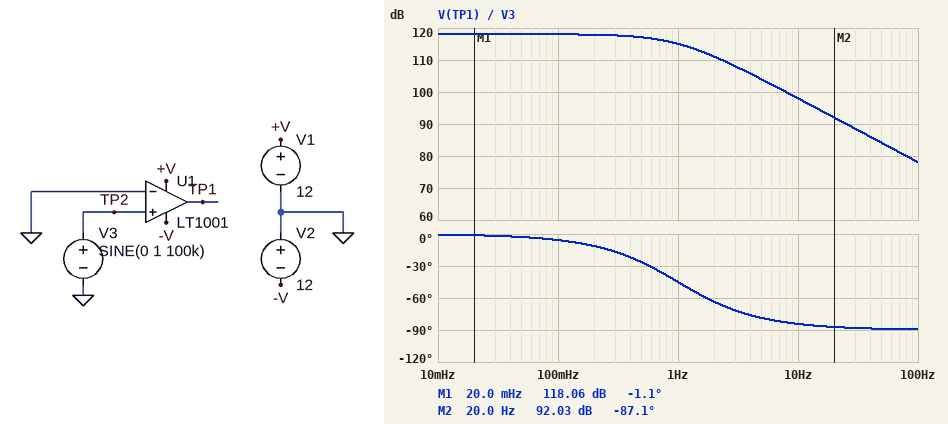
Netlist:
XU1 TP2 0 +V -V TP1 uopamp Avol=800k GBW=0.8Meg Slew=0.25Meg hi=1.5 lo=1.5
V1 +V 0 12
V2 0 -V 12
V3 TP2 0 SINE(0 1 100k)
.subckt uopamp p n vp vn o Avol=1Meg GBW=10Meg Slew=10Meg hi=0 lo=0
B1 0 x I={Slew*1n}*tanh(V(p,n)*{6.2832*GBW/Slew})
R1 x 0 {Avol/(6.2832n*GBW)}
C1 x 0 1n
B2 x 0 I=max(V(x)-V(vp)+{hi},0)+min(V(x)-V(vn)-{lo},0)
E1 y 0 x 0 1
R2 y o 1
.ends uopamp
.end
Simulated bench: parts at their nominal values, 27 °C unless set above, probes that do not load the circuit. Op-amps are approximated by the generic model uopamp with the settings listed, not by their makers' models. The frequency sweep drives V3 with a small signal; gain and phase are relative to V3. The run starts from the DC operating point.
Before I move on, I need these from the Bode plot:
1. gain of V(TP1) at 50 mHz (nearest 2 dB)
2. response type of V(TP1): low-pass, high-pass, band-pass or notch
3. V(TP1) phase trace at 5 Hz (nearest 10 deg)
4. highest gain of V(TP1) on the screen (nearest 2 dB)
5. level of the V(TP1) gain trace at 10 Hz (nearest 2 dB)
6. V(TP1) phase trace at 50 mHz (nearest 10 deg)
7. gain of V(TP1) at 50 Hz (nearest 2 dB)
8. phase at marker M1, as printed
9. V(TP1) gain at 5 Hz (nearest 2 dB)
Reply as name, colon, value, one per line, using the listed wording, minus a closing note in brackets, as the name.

gain of V(TP1) at 50 mHz: 118 dB
response type of V(TP1): low-pass, high-pass, band-pass or notch: low-pass
V(TP1) phase trace at 5 Hz: -80 deg
highest gain of V(TP1) on the screen: 118 dB
level of the V(TP1) gain trace at 10 Hz: 98 dB
V(TP1) phase trace at 50 mHz: 0 deg
gain of V(TP1) at 50 Hz: 84 dB
phase at marker M1, as printed: -1.1 deg
V(TP1) gain at 5 Hz: 104 dB
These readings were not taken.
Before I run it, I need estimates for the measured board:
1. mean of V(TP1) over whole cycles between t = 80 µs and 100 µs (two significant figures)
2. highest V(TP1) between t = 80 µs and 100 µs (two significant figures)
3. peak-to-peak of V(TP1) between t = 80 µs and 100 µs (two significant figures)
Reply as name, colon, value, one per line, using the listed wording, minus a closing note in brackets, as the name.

mean of V(TP1) over whole cycles between t = 80 µs and 100 µs: 610 mV
highest V(TP1) between t = 80 µs and 100 µs: 1.2 V
peak-to-peak of V(TP1) between t = 80 µs and 100 µs: 1.2 V
